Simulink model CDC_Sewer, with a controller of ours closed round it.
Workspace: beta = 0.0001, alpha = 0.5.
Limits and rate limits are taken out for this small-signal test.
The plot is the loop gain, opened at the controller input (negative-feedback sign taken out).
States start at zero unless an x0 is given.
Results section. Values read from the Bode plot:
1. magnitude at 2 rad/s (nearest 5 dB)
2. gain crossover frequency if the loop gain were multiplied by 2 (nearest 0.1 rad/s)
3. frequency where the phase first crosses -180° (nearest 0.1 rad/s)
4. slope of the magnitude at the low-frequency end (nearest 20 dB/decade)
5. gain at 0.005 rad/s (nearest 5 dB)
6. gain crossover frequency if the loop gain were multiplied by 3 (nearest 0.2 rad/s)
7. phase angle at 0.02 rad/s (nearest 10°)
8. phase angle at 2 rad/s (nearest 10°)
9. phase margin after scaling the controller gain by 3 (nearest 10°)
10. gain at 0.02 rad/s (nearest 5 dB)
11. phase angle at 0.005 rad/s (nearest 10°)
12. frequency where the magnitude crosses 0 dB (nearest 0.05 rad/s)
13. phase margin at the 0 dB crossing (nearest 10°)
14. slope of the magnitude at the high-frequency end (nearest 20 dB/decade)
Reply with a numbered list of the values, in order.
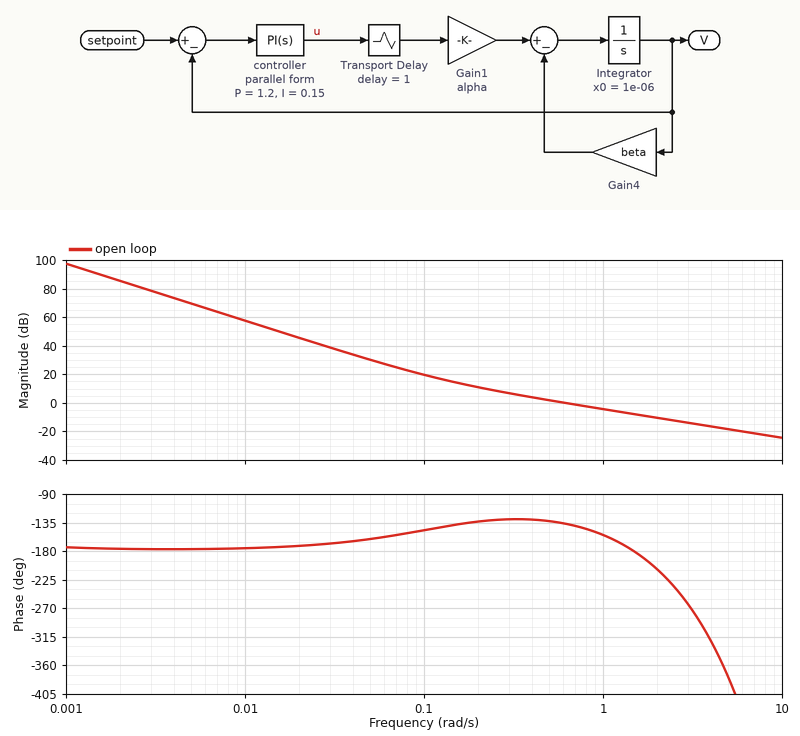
1. -10 dB
2. 1.2 rad/s
3. 1.5 rad/s
4. -40 dB/decade
5. 70 dB
6. 1.8 rad/s
7. -170°
8. -210°
9. -20°
10. 45 dB
11. -180°
12. 0.60 rad/s
13. 40°
14. -20 dB/decade
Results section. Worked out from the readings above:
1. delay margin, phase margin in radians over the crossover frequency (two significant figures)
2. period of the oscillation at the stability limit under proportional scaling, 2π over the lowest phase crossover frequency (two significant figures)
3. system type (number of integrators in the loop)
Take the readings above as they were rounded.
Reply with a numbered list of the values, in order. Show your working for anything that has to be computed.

1. 40 × π / 180 / 0.6 = 1.2 s
2. 2π / 1.5 = 4.2 s
3. 2
